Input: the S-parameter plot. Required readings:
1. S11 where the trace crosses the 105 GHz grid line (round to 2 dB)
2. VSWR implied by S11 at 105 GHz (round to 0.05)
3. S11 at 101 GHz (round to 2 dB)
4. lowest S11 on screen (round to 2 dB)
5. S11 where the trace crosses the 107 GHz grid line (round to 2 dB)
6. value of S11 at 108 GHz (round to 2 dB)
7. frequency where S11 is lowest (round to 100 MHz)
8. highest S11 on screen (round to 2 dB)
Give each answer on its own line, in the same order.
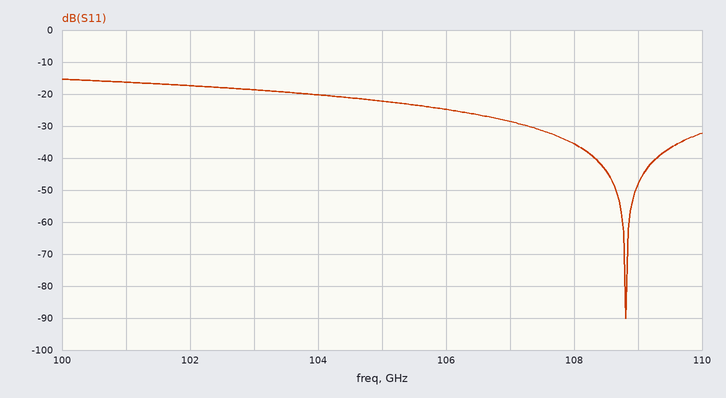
-22 dB
1.15
-16 dB
-90 dB
-28 dB
-36 dB
108.8 GHz
-16 dB
